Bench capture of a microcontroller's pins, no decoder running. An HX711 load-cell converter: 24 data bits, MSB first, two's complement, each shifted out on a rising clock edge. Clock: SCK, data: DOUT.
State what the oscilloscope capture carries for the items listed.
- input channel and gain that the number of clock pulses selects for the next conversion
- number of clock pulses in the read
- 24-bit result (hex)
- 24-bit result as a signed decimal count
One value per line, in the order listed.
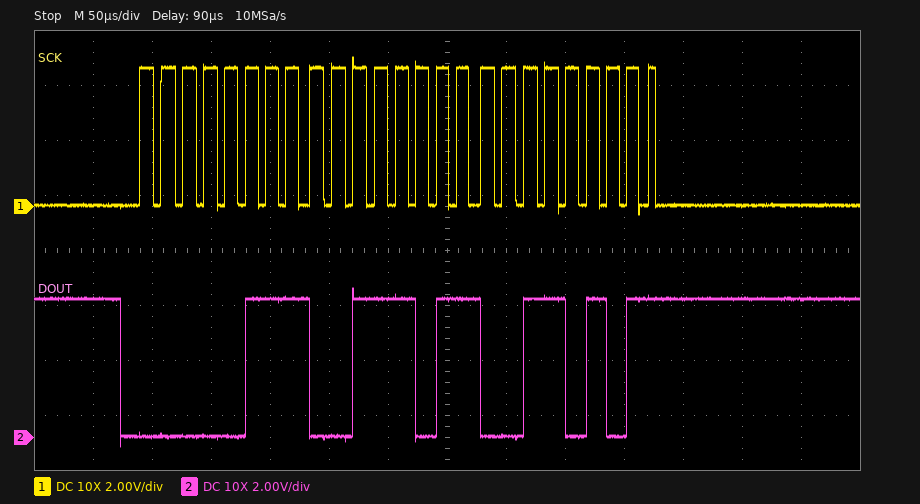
channel A, gain 128
25
0x073B35
473909
